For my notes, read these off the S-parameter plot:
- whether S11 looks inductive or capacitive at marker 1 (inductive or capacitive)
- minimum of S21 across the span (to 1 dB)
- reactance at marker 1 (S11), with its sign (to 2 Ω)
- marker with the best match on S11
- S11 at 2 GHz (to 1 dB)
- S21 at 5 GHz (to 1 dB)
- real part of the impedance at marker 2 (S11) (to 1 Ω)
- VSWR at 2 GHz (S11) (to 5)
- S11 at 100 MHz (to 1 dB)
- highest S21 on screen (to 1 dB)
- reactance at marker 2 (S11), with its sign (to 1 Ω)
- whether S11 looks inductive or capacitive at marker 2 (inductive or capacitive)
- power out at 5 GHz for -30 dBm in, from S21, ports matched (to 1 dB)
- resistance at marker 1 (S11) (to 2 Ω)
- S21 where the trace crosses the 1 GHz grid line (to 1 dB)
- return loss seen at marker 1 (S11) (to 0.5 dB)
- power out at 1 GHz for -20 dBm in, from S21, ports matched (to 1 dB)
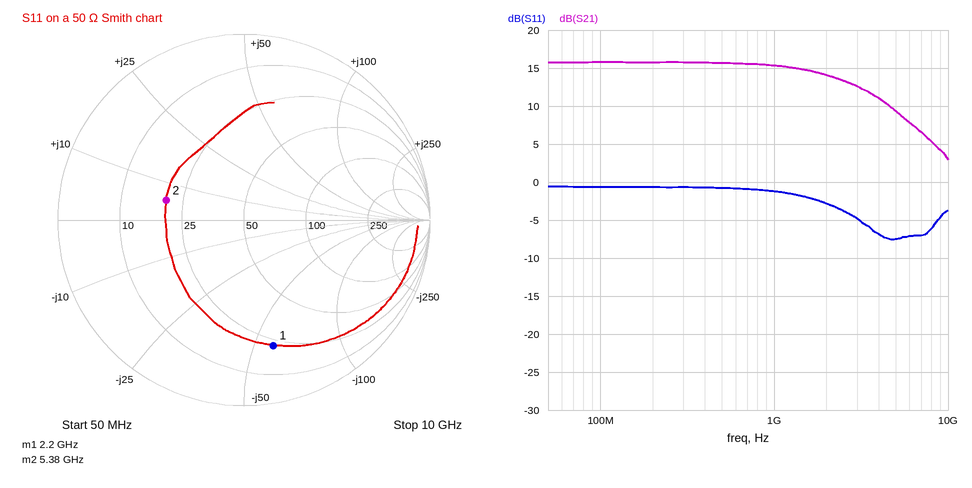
capacitive
3 dB
-58 Ω
marker 2
-3 dB
9 dB
20 Ω
5
-1 dB
16 dB
+5 Ω
inductive
-21 dBm
22 Ω
15 dB
3.0 dB
-5 dBm
